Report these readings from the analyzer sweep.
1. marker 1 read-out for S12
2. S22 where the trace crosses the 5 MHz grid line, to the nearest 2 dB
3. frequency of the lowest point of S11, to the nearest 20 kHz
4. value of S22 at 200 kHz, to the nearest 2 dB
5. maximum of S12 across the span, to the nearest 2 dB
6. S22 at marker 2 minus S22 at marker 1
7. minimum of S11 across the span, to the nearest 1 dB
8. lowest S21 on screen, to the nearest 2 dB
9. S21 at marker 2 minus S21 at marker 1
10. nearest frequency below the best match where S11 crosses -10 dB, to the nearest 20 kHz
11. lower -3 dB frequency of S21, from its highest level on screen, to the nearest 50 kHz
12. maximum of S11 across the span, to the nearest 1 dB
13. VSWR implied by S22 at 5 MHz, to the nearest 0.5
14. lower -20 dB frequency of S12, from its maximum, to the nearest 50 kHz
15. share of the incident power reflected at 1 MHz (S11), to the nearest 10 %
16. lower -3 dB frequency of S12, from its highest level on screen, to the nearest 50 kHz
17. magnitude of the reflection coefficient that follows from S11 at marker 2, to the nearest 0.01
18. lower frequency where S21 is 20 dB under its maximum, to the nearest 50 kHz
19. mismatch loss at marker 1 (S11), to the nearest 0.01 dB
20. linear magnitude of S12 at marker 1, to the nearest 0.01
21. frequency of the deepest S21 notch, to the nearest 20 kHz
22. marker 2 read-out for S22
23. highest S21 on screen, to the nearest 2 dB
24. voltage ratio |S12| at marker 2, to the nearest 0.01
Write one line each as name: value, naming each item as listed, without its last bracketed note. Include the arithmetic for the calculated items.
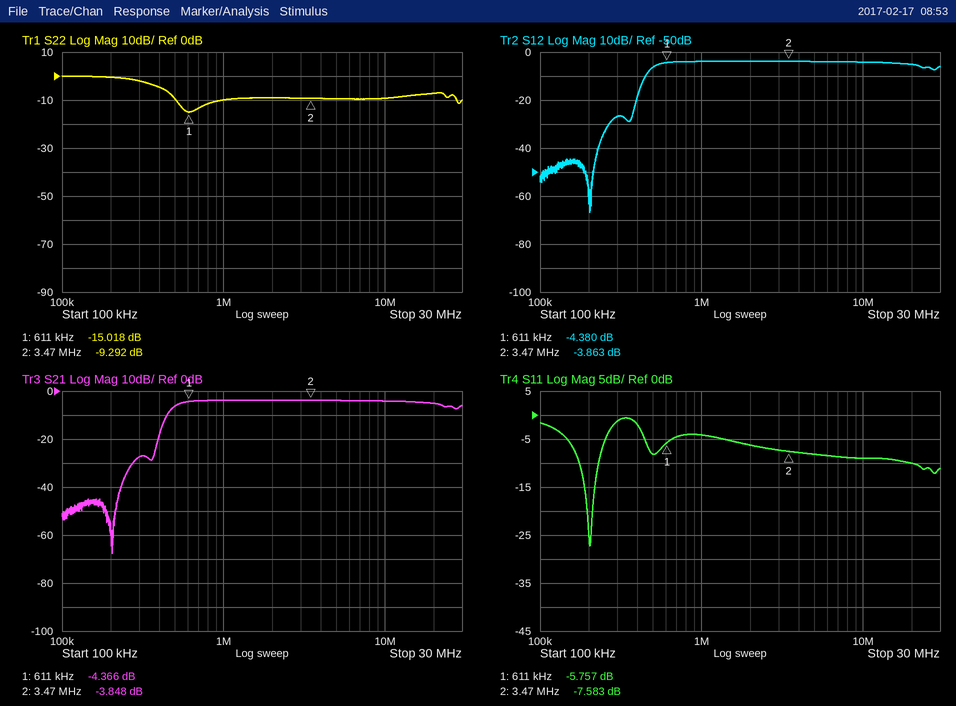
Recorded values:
marker 1 read-out for S12: -4.380 dB
S22 where the trace crosses the 5 MHz grid line, to the nearest 2 dB: -10 dB
frequency of the lowest point of S11, to the nearest 20 kHz: 200 kHz
value of S22 at 200 kHz, to the nearest 2 dB: 0 dB
maximum of S12 across the span, to the nearest 2 dB: -4 dB
S22 at marker 2 minus S22 at marker 1: -9.292 − (-15.018) = 5.726 dB
minimum of S11 across the span, to the nearest 1 dB: -27 dB
lowest S21 on screen, to the nearest 2 dB: -68 dB
S21 at marker 2 minus S21 at marker 1: -3.848 − (-4.366) = 0.518 dB
nearest frequency below the best match where S11 crosses -10 dB, to the nearest 20 kHz: 180 kHz
lower -3 dB frequency of S21, from its highest level on screen, to the nearest 50 kHz: 500 kHz
maximum of S11 across the span, to the nearest 1 dB: -1 dB
VSWR implied by S22 at 5 MHz, to the nearest 0.5: |Γ| = 10^(-10/20) = 0.3162; VSWR = (1 + 0.3162)/(1 − 0.3162) ≈ 1.92, so 2.0 to the nearest 0.5
lower -20 dB frequency of S12, from its maximum, to the nearest 50 kHz: 400 kHz
share of the incident power reflected at 1 MHz (S11), to the nearest 10 %: 10^(-4/10) ≈ 40 %
lower -3 dB frequency of S12, from its highest level on screen, to the nearest 50 kHz: 500 kHz
magnitude of the reflection coefficient that follows from S11 at marker 2, to the nearest 0.01: 10^(-7.583/20) ≈ 0.42
lower frequency where S21 is 20 dB under its maximum, to the nearest 50 kHz: 400 kHz
mismatch loss at marker 1 (S11), to the nearest 0.01 dB: −10 log10(1 − 10^(-5.757/10)) ≈ 1.34 dB
linear magnitude of S12 at marker 1, to the nearest 0.01: 10^(-4.38/20) ≈ 0.60
frequency of the deepest S21 notch, to the nearest 20 kHz: 200 kHz
marker 2 read-out for S22: -9.292 dB
highest S21 on screen, to the nearest 2 dB: -4 dB
voltage ratio |S12| at marker 2, to the nearest 0.01: 10^(-3.863/20) ≈ 0.64
